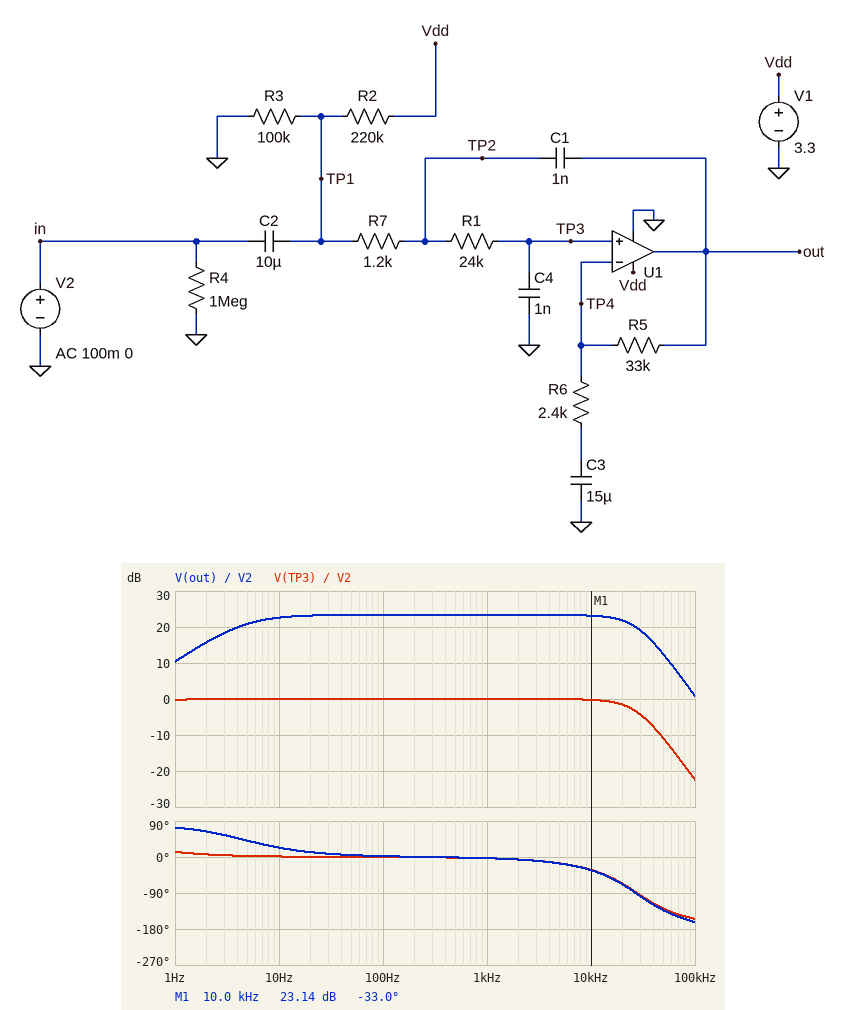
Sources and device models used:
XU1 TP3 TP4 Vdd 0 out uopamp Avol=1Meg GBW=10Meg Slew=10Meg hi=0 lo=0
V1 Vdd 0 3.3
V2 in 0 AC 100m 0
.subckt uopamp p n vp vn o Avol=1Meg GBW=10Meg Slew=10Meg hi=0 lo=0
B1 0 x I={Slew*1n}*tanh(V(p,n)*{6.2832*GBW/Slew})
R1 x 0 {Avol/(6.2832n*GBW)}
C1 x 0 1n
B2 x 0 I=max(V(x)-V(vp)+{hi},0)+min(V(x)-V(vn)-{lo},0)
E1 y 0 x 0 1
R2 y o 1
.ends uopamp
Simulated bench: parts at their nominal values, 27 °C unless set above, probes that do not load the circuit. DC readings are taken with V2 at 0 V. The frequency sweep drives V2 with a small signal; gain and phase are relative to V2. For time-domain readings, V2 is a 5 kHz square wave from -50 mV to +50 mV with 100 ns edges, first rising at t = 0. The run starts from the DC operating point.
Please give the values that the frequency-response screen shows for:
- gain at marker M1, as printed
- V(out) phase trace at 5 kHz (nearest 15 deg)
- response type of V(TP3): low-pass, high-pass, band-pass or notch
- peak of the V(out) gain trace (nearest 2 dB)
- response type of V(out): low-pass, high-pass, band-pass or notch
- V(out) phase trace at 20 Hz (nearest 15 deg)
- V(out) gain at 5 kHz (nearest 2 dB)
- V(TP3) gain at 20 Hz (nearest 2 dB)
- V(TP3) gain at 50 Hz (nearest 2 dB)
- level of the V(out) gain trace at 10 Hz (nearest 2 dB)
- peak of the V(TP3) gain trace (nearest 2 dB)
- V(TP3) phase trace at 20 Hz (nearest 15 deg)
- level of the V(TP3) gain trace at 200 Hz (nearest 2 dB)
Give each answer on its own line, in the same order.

23.14 dB
-15 deg
low-pass
24 dB
band-pass
15 deg
24 dB
0 dB
0 dB
22 dB
0 dB
0 deg
0 dB
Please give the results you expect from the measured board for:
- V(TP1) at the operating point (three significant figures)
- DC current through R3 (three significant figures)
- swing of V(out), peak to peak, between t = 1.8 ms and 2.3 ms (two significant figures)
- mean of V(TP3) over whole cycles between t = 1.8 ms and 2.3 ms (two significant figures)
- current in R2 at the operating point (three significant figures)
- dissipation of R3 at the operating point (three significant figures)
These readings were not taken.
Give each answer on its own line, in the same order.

1.03 V
10.3 µA
1.6 V
1.1 V
10.3 µA
10.6 µW
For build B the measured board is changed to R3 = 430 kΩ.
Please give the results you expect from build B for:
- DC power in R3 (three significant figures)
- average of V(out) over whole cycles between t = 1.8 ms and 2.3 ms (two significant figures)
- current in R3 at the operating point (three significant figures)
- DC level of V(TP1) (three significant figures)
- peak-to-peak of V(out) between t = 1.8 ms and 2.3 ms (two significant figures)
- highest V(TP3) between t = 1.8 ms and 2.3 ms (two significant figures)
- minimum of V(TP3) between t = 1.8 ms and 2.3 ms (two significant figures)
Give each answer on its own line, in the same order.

11.1 µW
2.8 V
5.08 µA
2.18 V
1.2 V
2.3 V
2.2 V
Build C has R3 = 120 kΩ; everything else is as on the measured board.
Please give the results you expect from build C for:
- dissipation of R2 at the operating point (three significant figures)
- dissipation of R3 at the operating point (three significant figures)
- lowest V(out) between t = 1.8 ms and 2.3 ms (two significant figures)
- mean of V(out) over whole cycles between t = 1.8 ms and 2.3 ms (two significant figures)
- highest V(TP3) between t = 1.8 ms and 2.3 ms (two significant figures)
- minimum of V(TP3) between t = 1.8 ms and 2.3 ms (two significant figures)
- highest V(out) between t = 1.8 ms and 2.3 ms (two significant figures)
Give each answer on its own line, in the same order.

20.7 µW
11.3 µW
1.1 V
1.9 V
1.3 V
1.2 V
2.6 V
